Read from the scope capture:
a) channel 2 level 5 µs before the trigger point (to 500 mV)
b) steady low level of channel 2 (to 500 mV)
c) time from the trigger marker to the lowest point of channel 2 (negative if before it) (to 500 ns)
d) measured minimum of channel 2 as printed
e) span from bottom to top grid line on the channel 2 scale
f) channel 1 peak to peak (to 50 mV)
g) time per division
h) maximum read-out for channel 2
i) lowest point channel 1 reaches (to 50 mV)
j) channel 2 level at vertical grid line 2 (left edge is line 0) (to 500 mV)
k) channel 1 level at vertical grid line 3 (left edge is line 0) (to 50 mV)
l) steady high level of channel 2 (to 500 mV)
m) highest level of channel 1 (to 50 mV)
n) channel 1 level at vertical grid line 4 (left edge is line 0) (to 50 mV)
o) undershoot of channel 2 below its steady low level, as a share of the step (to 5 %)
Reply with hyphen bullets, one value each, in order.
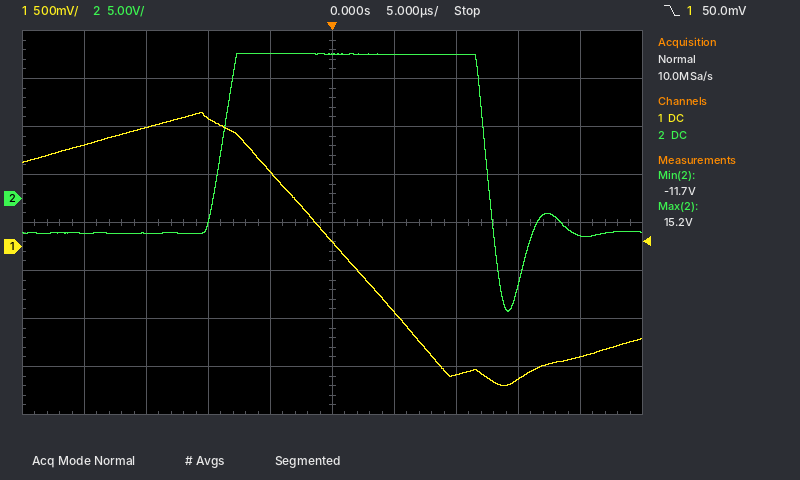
- 15.0 V
- -3.5 V
- +14.0 µs
- -11.7 V
- 40 V
- 2.85 V
- 5 µs
- 15.2 V
- -1.45 V
- -3.5 V
- 1.35 V
- 15.0 V
- 1.40 V
- 800 mV
- 45 %
